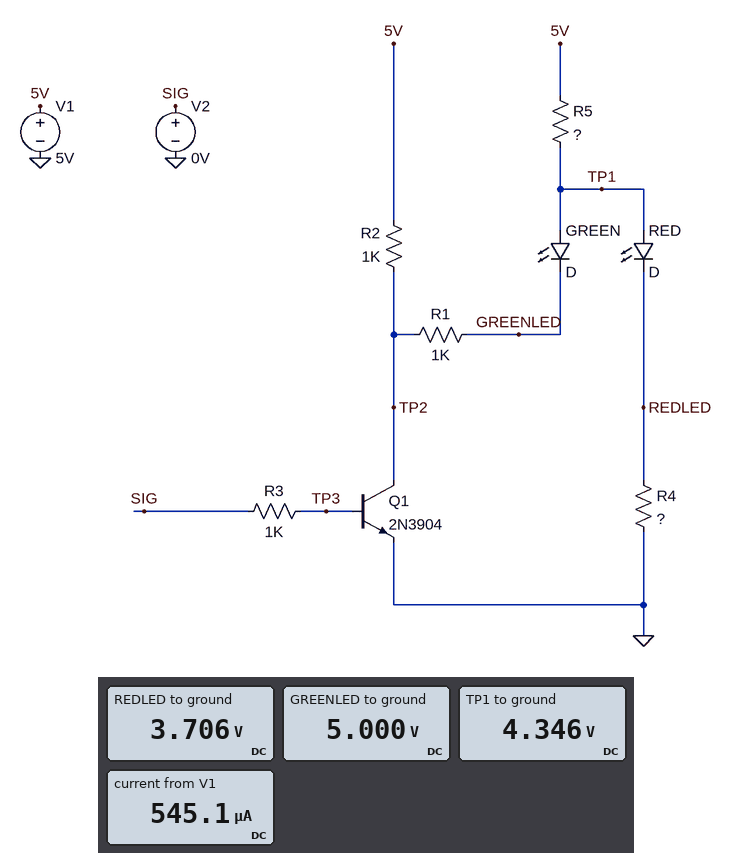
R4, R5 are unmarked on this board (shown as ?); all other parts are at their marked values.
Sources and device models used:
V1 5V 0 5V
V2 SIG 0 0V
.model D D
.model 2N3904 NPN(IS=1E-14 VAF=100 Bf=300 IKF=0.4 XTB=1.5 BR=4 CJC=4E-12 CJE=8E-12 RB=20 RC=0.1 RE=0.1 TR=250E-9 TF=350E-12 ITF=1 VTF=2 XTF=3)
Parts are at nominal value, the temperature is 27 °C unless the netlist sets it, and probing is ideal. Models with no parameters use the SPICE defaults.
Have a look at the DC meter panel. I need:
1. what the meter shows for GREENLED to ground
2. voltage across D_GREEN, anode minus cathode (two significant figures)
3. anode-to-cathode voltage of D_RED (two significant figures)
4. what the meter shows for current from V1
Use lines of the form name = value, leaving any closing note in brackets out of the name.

what the meter shows for GREENLED to ground = 5.000 V
voltage across D_GREEN, anode minus cathode = -650 mV
anode-to-cathode voltage of D_RED = 640 mV
what the meter shows for current from V1 = 545.1 µA
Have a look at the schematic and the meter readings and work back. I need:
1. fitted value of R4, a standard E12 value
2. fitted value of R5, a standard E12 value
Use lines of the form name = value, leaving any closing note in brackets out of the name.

fitted value of R4, a standard E12 value = 6.8 kΩ
fitted value of R5, a standard E12 value = 1.2 kΩ
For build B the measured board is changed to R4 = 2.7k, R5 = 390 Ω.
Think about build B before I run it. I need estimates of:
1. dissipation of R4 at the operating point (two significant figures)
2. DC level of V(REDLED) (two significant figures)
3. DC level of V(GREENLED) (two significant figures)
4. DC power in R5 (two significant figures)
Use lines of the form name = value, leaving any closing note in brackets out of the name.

dissipation of R4 at the operating point = 5.3 mW
DC level of V(REDLED) = 3.8 V
DC level of V(GREENLED) = 5.0 V
DC power in R5 = 770 µW
